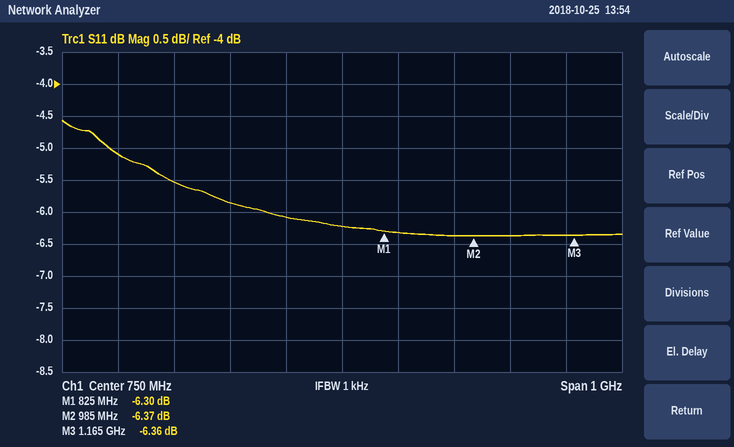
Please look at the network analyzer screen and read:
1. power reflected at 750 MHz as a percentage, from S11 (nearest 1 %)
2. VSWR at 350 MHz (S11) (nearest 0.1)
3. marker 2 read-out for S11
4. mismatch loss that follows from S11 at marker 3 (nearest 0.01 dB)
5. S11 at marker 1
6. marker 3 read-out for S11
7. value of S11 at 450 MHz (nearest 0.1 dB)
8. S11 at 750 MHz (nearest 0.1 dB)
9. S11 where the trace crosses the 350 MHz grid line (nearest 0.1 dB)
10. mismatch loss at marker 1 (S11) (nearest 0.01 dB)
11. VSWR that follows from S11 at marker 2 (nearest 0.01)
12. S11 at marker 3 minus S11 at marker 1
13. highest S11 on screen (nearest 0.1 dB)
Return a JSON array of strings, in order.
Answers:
["24 %", "3.5", "-6.37 dB", "1.14 dB", "-6.30 dB", "-6.36 dB", "-5.5 dB", "-6.2 dB", "-5.1 dB", "1.16 dB", "2.85", "-0.06 dB", "-4.6 dB"]
